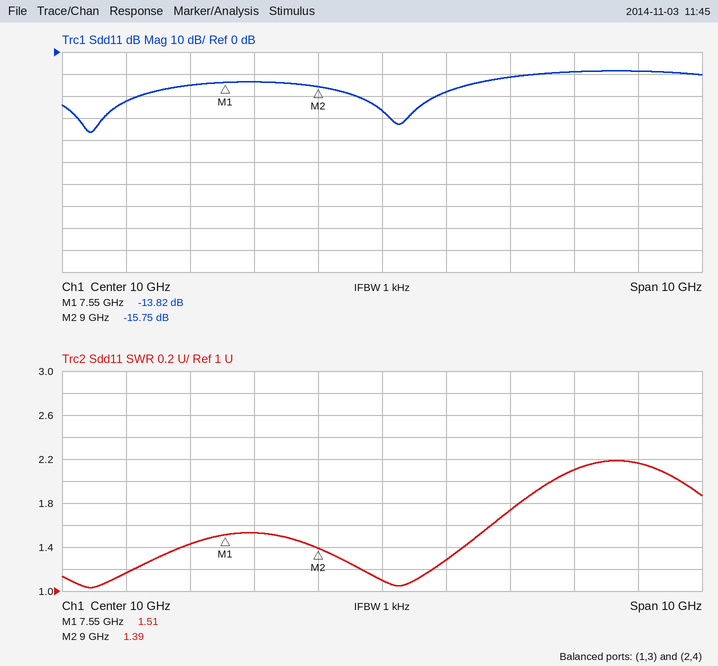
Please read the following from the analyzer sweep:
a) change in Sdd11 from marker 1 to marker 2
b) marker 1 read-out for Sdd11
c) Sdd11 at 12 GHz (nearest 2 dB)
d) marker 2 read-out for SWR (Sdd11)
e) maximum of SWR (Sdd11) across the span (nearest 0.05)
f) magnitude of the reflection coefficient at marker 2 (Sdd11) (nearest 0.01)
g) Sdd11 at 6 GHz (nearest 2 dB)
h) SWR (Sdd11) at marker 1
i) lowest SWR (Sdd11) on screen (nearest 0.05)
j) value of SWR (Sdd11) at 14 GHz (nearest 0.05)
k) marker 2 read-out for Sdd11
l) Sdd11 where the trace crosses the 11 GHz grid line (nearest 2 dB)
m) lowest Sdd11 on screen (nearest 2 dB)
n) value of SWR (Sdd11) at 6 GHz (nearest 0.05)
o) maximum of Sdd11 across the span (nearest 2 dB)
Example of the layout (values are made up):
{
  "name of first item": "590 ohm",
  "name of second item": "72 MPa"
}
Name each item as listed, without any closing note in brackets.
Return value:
{
  "change in Sdd11 from marker 1 to marker 2": "-1.93 dB",
  "marker 1 read-out for Sdd11": "-13.82 dB",
  "Sdd11 at 12 GHz": "-12 dB",
  "marker 2 read-out for SWR": "1.39",
  "maximum of SWR (Sdd11) across the span": "2.20",
  "magnitude of the reflection coefficient at marker 2 (Sdd11)": "0.16",
  "Sdd11 at 6 GHz": "-22 dB",
  "SWR (Sdd11) at marker 1": "1.51",
  "lowest SWR (Sdd11) on screen": "1.05",
  "value of SWR (Sdd11) at 14 GHz": "2.15",
  "marker 2 read-out for Sdd11": "-15.75 dB",
  "Sdd11 where the trace crosses the 11 GHz grid line": "-18 dB",
  "lowest Sdd11 on screen": "-36 dB",
  "value of SWR (Sdd11) at 6 GHz": "1.15",
  "maximum of Sdd11 across the span": "-8 dB"
}
